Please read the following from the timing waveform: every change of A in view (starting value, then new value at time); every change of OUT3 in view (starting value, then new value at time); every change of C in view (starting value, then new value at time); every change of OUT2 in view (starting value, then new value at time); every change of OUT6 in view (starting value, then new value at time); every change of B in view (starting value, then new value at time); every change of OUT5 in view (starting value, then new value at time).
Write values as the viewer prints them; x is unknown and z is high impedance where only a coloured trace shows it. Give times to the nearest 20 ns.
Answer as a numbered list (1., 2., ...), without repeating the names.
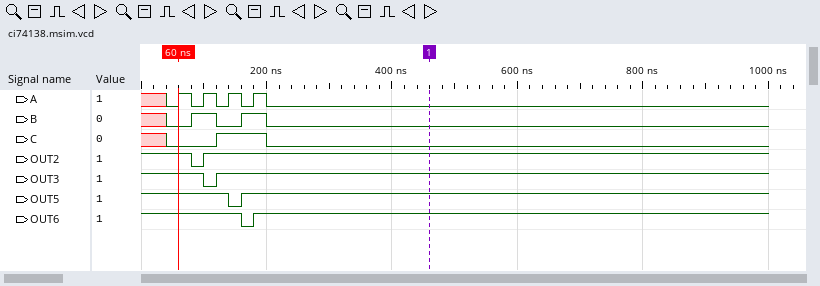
1. x, 0 at 40 ns, 1 at 60 ns, 0 at 80 ns, 1 at 100 ns, 0 at 120 ns, 1 at 140 ns, 0 at 160 ns, 1 at 180 ns, 0 at 200 ns
2. 1, 0 at 100 ns, 1 at 120 ns
3. x, 0 at 40 ns, 1 at 120 ns, 0 at 200 ns
4. 1, 0 at 80 ns, 1 at 100 ns
5. 1, 0 at 160 ns, 1 at 180 ns
6. x, 0 at 40 ns, 1 at 80 ns, 0 at 120 ns, 1 at 160 ns, 0 at 200 ns
7. 1, 0 at 140 ns, 1 at 160 ns
